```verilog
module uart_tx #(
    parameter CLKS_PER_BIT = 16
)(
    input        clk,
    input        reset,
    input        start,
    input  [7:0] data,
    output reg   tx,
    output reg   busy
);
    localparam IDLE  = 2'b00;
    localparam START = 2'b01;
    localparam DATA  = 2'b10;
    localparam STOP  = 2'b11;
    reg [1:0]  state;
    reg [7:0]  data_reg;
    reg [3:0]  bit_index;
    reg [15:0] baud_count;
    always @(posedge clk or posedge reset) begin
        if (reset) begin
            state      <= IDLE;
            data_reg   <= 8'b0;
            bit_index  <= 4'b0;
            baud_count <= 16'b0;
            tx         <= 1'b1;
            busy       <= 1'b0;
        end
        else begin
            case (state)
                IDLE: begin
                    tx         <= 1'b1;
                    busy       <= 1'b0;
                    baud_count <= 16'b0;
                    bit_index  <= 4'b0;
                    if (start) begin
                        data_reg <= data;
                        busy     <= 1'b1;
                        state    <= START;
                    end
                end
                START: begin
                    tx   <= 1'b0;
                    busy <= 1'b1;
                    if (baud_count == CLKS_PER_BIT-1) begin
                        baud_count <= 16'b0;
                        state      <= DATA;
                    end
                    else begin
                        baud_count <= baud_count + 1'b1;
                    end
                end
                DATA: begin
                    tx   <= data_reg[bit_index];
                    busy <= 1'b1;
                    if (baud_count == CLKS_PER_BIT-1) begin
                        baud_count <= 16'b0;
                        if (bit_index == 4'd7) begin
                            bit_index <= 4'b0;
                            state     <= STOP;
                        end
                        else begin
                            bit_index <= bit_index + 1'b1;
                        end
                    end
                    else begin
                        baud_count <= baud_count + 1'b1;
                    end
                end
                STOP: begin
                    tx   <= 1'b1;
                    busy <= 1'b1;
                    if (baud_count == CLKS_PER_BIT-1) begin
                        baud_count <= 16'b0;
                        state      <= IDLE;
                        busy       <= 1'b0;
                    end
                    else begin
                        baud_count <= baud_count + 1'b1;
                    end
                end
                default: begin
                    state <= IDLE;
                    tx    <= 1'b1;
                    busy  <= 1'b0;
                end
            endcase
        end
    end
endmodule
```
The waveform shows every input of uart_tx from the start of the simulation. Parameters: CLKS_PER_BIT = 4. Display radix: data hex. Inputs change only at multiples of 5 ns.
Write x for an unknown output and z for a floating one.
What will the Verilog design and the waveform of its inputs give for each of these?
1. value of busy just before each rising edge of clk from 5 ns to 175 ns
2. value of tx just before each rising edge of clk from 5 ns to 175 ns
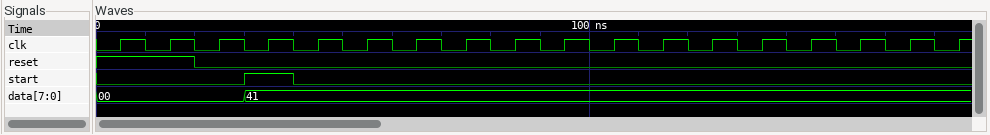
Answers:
0 0 0 0 1 1 1 1 1 1 1 1 1 1 1 1 1 1
1 1 1 1 1 0 0 0 0 1 1 1 1 0 0 0 0 0
